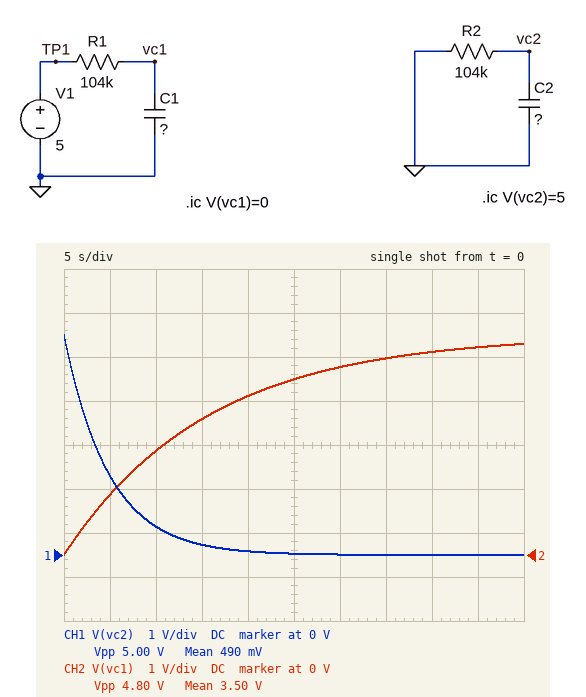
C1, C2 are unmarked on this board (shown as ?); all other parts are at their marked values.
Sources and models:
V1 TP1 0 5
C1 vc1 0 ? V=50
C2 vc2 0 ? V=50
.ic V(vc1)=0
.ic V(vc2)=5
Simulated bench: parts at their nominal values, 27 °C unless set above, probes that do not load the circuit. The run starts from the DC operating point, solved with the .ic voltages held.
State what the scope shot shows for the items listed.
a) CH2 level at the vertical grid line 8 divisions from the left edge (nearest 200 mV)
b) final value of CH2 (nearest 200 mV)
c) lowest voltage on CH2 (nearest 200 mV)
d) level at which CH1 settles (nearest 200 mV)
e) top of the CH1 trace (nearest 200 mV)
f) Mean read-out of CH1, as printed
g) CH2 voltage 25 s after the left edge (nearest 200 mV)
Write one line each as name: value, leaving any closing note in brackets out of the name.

CH2 level at the vertical grid line 8 divisions from the left edge: 4.6 V
final value of CH2: 4.8 V
lowest voltage on CH2: 0 V
level at which CH1 settles: 0 V
top of the CH1 trace: 5.0 V
Mean read-out of CH1, as printed: 490 mV
CH2 voltage 25 s after the left edge: 4.0 V
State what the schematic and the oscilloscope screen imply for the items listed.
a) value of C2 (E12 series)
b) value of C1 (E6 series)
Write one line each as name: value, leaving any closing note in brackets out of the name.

value of C2: 47 µF
value of C1: 150 µF
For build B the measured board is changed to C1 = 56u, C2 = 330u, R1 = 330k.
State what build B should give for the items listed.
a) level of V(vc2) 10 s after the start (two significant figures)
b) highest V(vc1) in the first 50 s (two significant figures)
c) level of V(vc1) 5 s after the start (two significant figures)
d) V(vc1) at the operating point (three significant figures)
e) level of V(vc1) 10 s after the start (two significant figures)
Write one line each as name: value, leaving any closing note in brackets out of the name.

level of V(vc2) 10 s after the start: 3.7 V
highest V(vc1) in the first 50 s: 4.7 V
level of V(vc1) 5 s after the start: 1.2 V
V(vc1) at the operating point: 5.00 V
level of V(vc1) 10 s after the start: 2.1 V
